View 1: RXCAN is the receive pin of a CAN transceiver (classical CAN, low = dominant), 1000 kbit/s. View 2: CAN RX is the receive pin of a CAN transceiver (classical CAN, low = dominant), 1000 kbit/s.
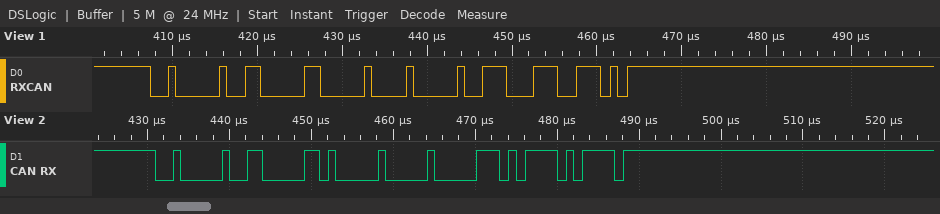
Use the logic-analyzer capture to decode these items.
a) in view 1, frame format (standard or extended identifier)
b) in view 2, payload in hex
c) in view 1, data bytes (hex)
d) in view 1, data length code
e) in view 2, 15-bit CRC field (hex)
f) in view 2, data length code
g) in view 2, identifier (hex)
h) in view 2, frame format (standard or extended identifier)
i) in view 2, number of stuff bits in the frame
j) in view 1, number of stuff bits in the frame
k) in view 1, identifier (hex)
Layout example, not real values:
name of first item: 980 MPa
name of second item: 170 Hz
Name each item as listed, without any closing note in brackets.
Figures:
in view 1, frame format: standard
in view 2, payload in hex: 80 00
in view 1, data bytes: 00 80
in view 1, data length code: 2
in view 2, 15-bit CRC field: 0x6BD7
in view 2, data length code: 2
in view 2, identifier: 0x203
in view 2, frame format: standard
in view 2, number of stuff bits in the frame: 5
in view 1, number of stuff bits in the frame: 4
in view 1, identifier: 0x203
